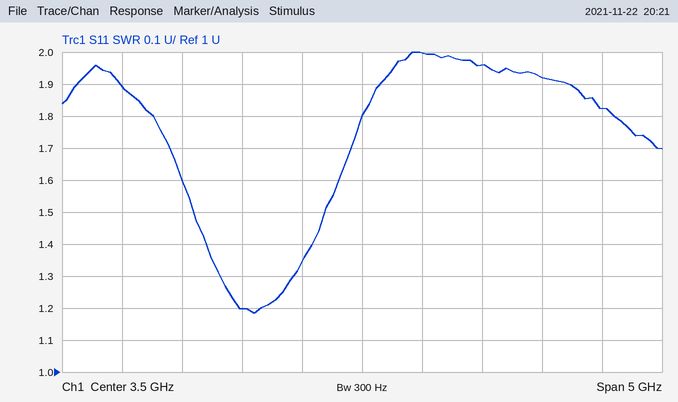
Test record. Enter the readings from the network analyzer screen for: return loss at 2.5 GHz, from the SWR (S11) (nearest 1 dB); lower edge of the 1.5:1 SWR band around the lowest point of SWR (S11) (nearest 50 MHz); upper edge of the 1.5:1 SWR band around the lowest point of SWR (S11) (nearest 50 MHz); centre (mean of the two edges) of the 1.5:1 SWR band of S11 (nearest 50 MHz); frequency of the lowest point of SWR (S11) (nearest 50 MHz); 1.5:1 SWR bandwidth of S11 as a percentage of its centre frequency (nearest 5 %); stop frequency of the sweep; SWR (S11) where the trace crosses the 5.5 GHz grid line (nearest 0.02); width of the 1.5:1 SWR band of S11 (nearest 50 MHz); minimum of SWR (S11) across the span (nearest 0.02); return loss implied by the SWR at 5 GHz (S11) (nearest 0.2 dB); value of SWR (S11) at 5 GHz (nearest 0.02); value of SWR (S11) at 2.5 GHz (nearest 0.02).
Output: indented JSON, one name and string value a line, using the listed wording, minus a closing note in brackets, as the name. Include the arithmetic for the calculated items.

{
  "return loss at 2.5 GHz, from the SWR (S11)": "−20 log10((1.2 − 1)/(1.2 + 1)) ≈ 21 dB",
  "lower edge of the 1.5:1 SWR band around the lowest point of SWR (S11)": "2.10 GHz",
  "upper edge of the 1.5:1 SWR band around the lowest point of SWR (S11)": "3.20 GHz",
  "centre (mean of the two edges) of the 1.5:1 SWR band of S11": "2.65 GHz",
  "frequency of the lowest point of SWR (S11)": "2.60 GHz",
  "1.5:1 SWR bandwidth of S11 as a percentage of its centre frequency": "1.1 GHz / 2.65 GHz ≈ 41.5 %, so 40 % to the nearest 5 %",
  "stop frequency of the sweep": "6 GHz",
  "SWR (S11) where the trace crosses the 5.5 GHz grid line": "1.82",
  "width of the 1.5:1 SWR band of S11": "3.20 GHz − 2.10 GHz = 1.10 GHz",
  "minimum of SWR (S11) across the span": "1.18",
  "return loss implied by the SWR at 5 GHz (S11)": "−20 log10((1.92 − 1)/(1.92 + 1)) ≈ 10.0 dB",
  "value of SWR (S11) at 5 GHz": "1.92",
  "value of SWR (S11) at 2.5 GHz": "1.20"
}
